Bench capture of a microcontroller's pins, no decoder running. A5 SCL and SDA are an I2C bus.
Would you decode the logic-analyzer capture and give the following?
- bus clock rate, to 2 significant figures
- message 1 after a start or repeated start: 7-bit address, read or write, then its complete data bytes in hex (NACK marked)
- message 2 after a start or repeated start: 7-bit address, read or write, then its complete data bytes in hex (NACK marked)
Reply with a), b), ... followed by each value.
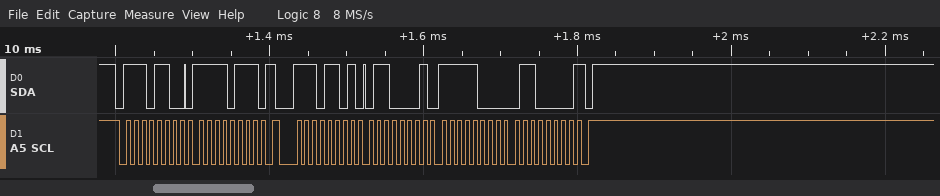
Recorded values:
a) 100 kHz
b) 0x76 write: F7
c) 0x76 read: 61 F8 60 NACK
